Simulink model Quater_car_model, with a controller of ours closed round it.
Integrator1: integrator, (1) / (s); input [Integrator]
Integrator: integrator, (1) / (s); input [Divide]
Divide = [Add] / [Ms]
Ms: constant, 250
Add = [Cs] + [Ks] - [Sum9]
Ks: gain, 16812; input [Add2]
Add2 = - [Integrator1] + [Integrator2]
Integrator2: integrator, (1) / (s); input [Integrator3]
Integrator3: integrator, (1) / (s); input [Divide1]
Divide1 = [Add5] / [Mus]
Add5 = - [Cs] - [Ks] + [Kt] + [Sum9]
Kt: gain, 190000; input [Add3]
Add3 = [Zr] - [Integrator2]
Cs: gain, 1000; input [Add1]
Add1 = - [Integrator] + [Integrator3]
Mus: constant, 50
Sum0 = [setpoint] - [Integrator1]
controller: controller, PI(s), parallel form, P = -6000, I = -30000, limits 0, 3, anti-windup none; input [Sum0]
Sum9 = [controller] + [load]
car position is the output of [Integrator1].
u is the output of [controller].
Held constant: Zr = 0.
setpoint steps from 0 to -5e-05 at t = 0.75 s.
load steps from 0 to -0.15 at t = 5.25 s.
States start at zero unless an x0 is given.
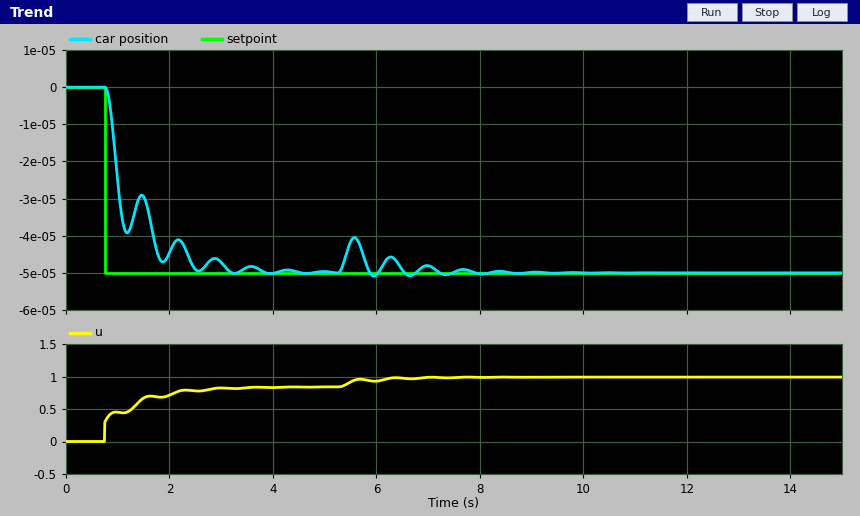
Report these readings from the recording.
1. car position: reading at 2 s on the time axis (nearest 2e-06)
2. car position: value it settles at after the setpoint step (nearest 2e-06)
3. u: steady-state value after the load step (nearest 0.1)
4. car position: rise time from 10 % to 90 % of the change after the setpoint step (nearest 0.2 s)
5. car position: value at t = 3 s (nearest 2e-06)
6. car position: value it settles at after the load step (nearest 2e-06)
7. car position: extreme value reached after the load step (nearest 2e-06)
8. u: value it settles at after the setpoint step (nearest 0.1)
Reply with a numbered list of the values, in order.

1. -0.000044
2. -0.000050
3. 1.0
4. 1.0 s
5. -0.000048
6. -0.000050
7. -0.000040
8. 0.8
